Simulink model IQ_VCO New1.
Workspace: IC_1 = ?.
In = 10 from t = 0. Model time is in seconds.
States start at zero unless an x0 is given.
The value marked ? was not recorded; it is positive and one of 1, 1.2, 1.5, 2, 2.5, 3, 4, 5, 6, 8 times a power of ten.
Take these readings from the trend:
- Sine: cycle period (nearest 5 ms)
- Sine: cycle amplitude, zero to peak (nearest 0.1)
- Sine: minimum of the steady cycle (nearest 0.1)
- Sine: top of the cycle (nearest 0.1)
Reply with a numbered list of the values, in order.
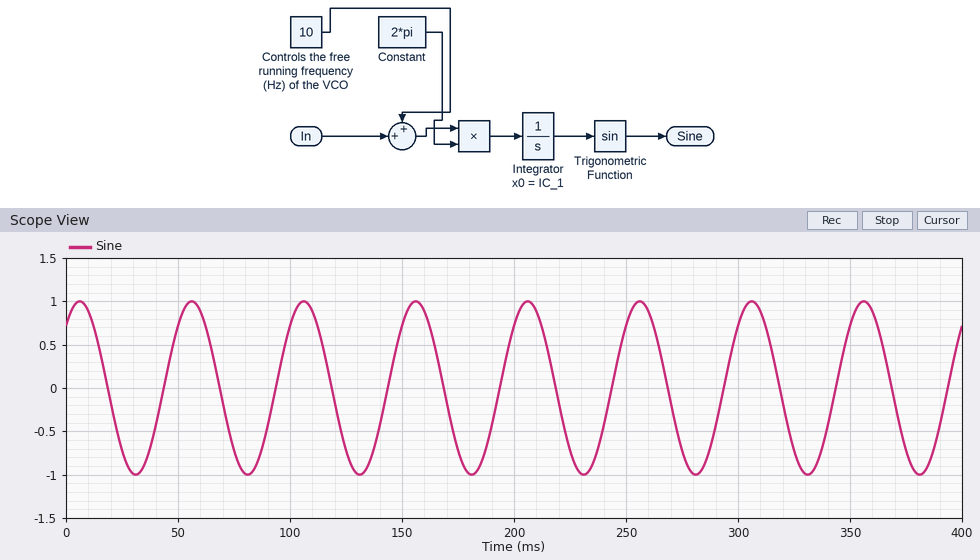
1. 50 ms
2. 1.0
3. -1.0
4. 1.0
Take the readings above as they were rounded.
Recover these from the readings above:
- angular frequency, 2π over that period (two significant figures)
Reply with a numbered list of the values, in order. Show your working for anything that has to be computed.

1. 2π / 50 = 0.13 rad/ms
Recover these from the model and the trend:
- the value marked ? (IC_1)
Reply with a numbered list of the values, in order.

1. 0.8
